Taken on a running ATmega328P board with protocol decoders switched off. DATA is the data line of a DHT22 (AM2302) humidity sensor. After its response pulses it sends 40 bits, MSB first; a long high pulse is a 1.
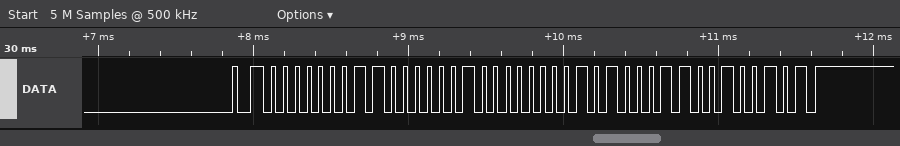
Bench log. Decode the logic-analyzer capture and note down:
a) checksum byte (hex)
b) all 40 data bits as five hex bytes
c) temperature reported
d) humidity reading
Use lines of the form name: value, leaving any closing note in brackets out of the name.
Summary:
checksum byte: 0x25
all 40 data bits as five hex bytes: 01 81 00 A3 25
temperature reported: 16.3 °C
humidity reading: 38.5 %
